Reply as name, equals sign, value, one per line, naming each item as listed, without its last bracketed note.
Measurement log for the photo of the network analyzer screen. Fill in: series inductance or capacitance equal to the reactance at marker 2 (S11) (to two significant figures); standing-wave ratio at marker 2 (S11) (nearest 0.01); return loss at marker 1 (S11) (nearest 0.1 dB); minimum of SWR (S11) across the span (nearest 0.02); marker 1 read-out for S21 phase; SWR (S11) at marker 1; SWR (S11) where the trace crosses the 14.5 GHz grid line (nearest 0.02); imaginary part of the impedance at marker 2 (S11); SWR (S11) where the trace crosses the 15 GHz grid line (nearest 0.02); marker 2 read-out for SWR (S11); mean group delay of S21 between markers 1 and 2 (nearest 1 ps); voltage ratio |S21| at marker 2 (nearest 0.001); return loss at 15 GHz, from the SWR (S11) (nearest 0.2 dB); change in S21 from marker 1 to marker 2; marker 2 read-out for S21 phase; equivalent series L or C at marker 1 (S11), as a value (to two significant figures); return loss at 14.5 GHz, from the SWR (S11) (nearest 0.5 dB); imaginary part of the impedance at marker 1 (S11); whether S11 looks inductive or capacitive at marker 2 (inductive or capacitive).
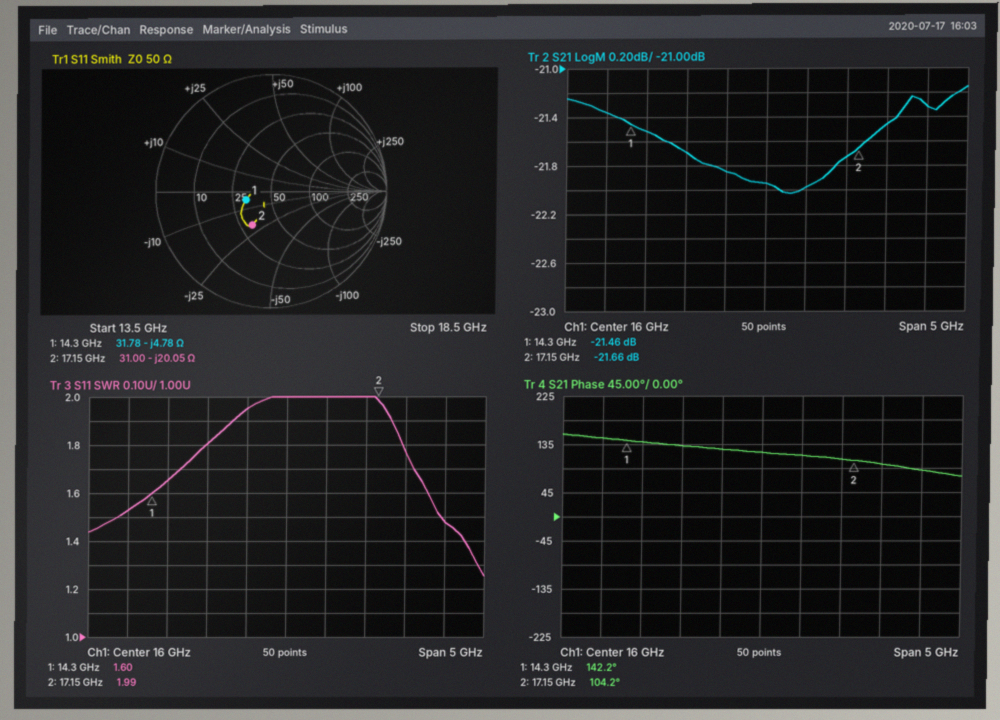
series inductance or capacitance equal to the reactance at marker 2 (S11) = 460 fF
standing-wave ratio at marker 2 (S11) = 1.99
return loss at marker 1 (S11) = 12.8 dB
minimum of SWR (S11) across the span = 1.26
marker 1 read-out for S21 phase = 142.2°
SWR (S11) at marker 1 = 1.60
SWR (S11) where the trace crosses the 14.5 GHz grid line = 1.66
imaginary part of the impedance at marker 2 = -20.05 Ω
SWR (S11) where the trace crosses the 15 GHz grid line = 1.80
marker 2 read-out for SWR = 1.99
mean group delay of S21 between markers 1 and 2 = 37 ps
voltage ratio |S21| at marker 2 = 0.083
return loss at 15 GHz, from the SWR (S11) = 10.8 dB
change in S21 from marker 1 to marker 2 = -0.20 dB
marker 2 read-out for S21 phase = 104.2°
equivalent series L or C at marker 1 (S11), as a value = 2.3 pF
return loss at 14.5 GHz, from the SWR (S11) = 12.0 dB
imaginary part of the impedance at marker 1 = -4.78 Ω
whether S11 looks inductive or capacitive at marker 2 = capacitive
